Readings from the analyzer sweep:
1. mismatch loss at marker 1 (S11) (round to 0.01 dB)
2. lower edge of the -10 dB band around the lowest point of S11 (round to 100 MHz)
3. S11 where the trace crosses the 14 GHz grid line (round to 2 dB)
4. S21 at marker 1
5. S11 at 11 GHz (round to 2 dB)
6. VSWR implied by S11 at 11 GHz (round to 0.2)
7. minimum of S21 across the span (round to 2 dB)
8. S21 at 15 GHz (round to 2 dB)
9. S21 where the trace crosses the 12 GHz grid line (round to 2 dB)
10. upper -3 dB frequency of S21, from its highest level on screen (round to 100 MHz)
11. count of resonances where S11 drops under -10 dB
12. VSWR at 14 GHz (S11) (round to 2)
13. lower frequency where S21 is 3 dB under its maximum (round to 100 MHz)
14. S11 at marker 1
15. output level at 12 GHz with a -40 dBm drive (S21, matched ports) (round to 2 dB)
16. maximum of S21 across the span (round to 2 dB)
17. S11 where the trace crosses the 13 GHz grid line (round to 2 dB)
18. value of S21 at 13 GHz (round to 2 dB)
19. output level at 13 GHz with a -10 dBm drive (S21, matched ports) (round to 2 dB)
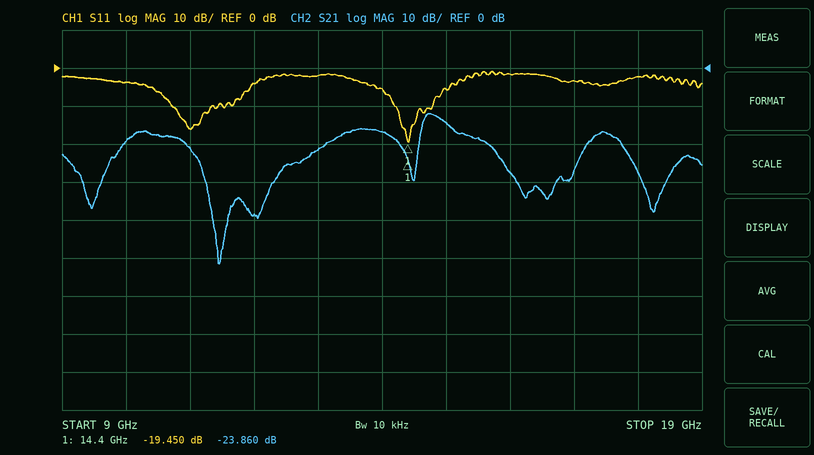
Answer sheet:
0.05 dB
14.2 GHz
-6 dB
-23.860 dB
-16 dB
1.4
-52 dB
-14 dB
-38 dB
15.0 GHz
2
4
14.6 GHz
-19.450 dB
-78 dBm
-12 dB
-2 dB
-22 dB
-32 dBm
